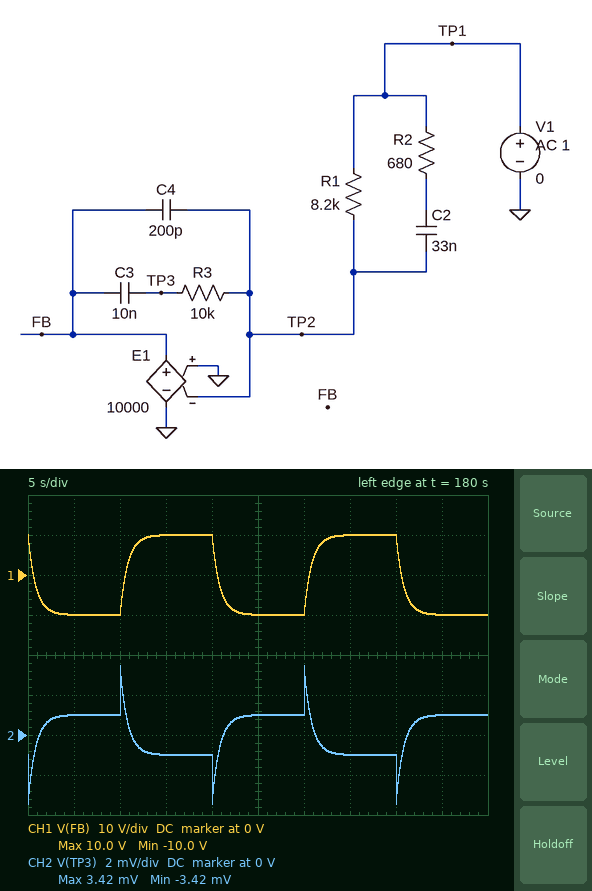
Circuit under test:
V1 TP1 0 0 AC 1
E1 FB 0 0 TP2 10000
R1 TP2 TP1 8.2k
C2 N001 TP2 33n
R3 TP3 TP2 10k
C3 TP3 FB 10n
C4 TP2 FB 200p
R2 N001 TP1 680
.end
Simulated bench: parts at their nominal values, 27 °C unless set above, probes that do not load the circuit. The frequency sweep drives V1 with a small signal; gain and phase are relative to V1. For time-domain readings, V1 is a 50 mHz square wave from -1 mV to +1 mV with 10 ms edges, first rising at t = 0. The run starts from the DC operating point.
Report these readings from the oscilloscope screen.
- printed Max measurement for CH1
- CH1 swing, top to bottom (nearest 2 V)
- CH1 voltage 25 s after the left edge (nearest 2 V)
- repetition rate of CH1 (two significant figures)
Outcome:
10.0 V
20 V
-10 V
50 mHz
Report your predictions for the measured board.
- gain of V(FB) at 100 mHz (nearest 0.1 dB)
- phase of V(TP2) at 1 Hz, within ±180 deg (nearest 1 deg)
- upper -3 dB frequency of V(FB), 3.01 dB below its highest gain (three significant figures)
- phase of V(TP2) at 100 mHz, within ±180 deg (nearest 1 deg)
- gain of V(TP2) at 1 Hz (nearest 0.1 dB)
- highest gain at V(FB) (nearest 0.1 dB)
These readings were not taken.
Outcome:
78.9 dB
-79 deg
190 mHz
-28 deg
-14.6 dB
80.0 dB
